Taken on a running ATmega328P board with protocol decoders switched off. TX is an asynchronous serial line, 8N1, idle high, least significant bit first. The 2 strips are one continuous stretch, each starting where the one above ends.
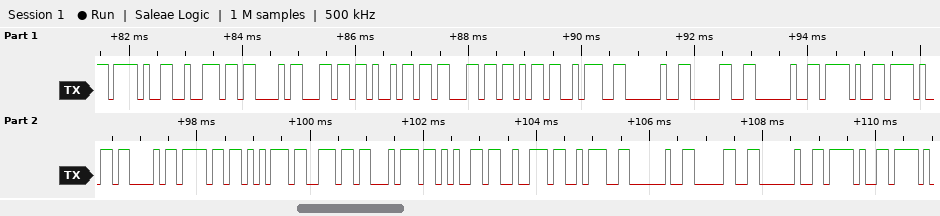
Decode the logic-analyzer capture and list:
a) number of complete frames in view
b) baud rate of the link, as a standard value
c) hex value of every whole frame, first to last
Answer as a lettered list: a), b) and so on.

a) 25
b) 9600 baud
c) 2F 72 43 6C 69 63 6B 3A 20 30 20 2F 2F 43 6F 75 6E 74 65 72 3A 20 30 20 2F
